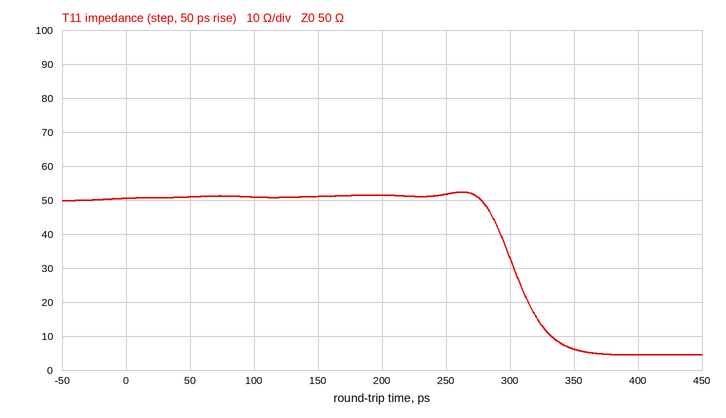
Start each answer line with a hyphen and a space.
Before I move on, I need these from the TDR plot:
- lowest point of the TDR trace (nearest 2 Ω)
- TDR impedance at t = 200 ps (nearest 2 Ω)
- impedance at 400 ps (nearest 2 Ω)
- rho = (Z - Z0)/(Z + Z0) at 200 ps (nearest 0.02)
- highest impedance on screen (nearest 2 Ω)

- 4 Ω
- 52 Ω
- 4 Ω
- +0.02
- 52 Ω
